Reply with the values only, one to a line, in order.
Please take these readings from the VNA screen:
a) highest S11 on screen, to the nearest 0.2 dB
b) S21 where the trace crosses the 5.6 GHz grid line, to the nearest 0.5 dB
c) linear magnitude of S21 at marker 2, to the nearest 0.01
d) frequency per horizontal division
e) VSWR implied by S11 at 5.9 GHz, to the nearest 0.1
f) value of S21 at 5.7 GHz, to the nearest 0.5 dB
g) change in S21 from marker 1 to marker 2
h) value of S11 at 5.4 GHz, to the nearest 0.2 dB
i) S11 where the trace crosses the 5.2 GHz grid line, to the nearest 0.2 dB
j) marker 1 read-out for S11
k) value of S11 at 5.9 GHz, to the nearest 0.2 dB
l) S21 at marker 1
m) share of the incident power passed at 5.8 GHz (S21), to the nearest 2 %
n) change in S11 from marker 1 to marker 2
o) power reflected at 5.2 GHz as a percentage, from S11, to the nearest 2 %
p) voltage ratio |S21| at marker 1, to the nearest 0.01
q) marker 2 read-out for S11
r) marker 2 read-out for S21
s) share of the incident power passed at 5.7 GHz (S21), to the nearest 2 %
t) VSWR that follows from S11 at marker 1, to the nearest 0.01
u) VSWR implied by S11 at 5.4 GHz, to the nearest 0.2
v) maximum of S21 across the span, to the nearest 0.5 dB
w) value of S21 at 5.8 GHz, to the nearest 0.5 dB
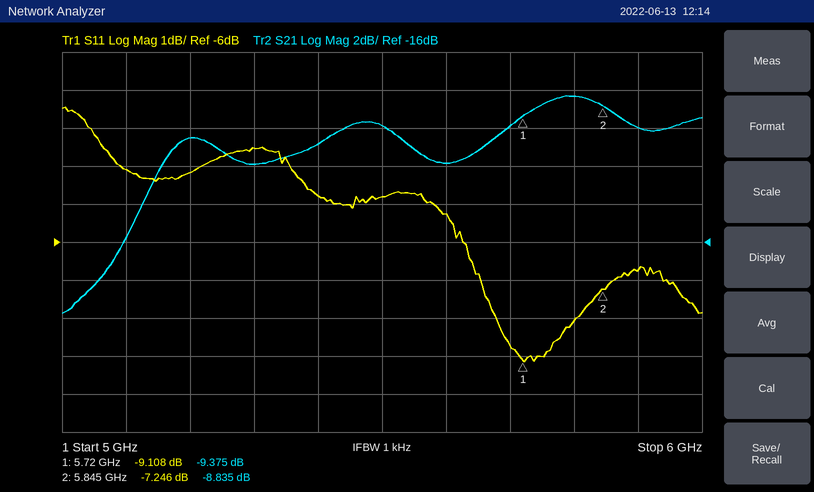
-2.4 dB
-12.0 dB
0.36
100 MHz
2.7
-10.0 dB
0.540 dB
-4.8 dB
-4.2 dB
-9.108 dB
-6.8 dB
-9.375 dB
14 %
1.862 dB
38 %
0.34
-7.246 dB
-8.835 dB
10 %
2.08
3.8
-8.5 dB
-8.5 dB
